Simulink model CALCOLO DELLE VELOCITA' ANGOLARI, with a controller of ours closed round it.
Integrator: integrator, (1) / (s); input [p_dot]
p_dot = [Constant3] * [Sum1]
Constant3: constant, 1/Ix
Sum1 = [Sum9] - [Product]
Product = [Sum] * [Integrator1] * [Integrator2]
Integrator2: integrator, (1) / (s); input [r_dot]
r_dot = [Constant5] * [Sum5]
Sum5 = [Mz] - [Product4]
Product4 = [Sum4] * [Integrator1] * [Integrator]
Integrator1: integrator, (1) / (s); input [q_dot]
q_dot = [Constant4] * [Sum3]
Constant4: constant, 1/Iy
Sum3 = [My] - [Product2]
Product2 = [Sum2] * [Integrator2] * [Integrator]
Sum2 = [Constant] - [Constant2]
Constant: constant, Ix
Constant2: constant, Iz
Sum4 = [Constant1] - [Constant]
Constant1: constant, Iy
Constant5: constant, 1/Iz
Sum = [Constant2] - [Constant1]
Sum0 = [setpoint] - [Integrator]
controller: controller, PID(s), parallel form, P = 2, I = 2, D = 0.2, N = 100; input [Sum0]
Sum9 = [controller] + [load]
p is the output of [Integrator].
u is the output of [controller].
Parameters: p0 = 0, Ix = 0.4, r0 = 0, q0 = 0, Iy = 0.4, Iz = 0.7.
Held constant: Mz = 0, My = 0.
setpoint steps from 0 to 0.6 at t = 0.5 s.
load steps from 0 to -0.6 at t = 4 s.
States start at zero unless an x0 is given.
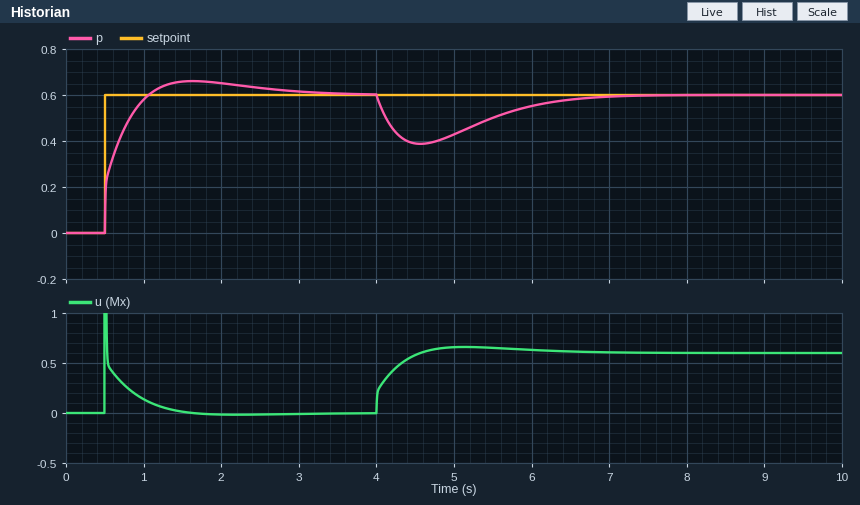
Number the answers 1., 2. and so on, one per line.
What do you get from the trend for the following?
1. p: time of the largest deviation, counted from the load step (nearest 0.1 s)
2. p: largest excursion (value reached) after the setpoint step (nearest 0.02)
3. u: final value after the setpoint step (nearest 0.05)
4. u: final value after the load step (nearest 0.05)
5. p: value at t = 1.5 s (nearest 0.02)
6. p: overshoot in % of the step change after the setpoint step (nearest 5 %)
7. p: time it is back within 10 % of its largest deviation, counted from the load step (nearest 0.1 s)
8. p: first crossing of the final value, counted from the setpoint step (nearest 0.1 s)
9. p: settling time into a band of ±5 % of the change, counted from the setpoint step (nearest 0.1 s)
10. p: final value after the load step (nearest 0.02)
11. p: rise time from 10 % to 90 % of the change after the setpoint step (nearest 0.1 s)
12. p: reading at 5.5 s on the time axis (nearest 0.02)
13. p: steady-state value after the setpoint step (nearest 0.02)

1. 0.6 s
2. 0.66
3. 0.00
4. 0.60
5. 0.66
6. 10 %
7. 2.5 s
8. 0.6 s
9. 2.0 s
10. 0.60
11. 0.4 s
12. 0.50
13. 0.60
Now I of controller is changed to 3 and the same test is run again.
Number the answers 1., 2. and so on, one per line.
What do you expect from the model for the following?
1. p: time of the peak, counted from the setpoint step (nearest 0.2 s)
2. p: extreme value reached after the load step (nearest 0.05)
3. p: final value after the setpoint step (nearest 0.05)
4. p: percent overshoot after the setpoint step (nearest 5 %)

1. 1.0 s
2. 0.40
3. 0.60
4. 15 %
